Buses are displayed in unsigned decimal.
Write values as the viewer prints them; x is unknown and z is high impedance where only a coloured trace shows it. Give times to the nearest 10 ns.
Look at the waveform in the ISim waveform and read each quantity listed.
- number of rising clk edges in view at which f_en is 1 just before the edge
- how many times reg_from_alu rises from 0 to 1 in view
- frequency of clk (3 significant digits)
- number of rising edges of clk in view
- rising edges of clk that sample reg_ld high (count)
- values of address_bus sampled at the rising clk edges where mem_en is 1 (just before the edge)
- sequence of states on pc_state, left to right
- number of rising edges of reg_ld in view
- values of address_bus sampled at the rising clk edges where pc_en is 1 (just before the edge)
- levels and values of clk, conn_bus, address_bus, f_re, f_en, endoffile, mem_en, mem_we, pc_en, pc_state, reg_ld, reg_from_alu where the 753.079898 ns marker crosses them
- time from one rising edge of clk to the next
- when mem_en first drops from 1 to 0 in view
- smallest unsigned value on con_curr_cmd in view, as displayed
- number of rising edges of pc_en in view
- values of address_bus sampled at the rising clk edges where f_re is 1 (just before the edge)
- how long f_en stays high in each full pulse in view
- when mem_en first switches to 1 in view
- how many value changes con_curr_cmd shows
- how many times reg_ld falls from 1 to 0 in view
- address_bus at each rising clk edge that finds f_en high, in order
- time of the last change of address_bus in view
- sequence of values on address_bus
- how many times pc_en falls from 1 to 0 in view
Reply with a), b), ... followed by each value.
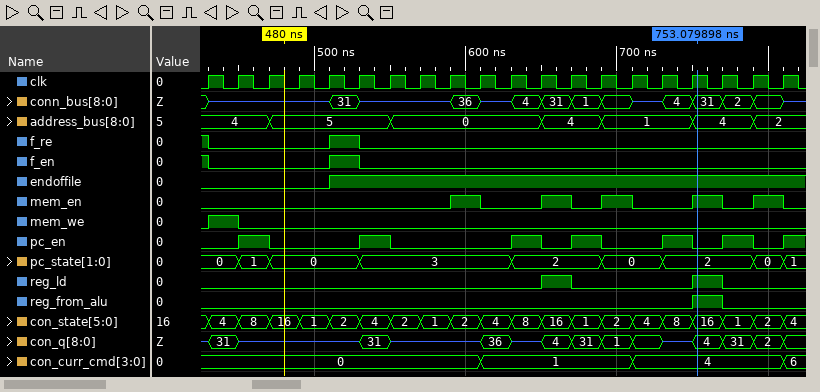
a) 2
b) 1
c) 50.0 MHz
d) 20
e) 2
f) 0, 4, 1, 4, 2
g) 0, 1, 0, 3, 2, 0, 2, 0, 1
h) 2
i) 4, 5, 0, 4, 1, 4
j) clk=1, conn_bus=31, address_bus=4, f_re=0, f_en=0, endoffile=1, mem_en=1, mem_we=0, pc_en=0, pc_state=2, reg_ld=1, reg_from_alu=1
k) 20 ns
l) 610 ns
m) 0
n) 7
o) 4, 5
p) 20 ns
q) 590 ns
r) 3
s) 2
t) 4, 5
u) 790 ns
v) 4, 5, 0, 4, 1, 4, 2
w) 6
